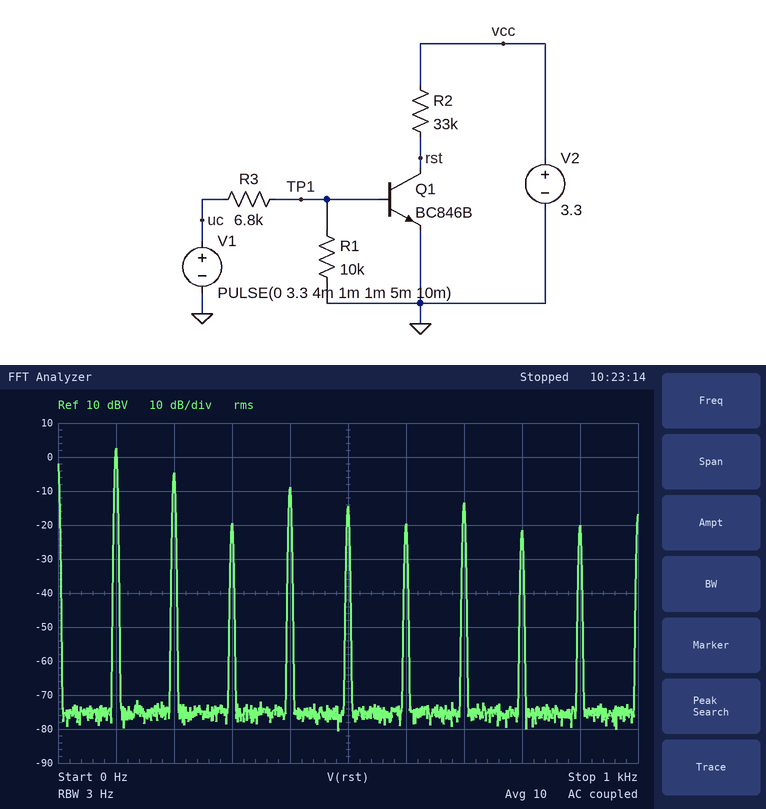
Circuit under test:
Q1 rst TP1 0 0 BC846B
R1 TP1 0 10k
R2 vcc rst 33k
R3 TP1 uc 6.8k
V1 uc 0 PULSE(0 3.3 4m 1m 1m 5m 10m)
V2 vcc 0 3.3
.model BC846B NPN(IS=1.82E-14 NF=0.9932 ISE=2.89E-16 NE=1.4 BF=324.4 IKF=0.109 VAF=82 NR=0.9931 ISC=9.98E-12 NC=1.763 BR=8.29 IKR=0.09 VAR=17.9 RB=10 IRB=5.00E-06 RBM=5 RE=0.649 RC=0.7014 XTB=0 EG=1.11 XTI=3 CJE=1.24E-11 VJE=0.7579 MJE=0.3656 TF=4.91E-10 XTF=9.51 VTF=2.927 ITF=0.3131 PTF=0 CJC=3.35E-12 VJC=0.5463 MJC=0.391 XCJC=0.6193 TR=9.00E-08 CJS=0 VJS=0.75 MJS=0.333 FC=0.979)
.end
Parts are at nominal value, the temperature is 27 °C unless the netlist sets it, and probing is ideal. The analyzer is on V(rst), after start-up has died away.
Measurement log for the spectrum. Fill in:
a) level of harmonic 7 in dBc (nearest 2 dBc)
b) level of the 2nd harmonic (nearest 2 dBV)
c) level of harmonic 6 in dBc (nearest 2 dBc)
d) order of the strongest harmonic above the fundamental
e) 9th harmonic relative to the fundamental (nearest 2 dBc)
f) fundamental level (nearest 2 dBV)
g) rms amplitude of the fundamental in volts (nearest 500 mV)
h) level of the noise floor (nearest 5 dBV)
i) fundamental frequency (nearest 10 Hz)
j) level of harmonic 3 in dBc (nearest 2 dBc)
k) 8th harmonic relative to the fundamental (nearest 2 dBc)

-16 dBc
-4 dBV
-22 dBc
2
-22 dBc
2 dBV
1.5 V
-75 dBV
100 Hz
-22 dBc
-24 dBc
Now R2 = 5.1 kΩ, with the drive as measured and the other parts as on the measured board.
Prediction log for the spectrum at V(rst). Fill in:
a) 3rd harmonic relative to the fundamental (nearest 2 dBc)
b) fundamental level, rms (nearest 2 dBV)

-20 dBc
2 dBV
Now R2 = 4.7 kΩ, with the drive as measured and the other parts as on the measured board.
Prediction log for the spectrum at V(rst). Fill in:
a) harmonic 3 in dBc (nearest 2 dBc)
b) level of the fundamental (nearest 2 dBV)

-20 dBc
2 dBV
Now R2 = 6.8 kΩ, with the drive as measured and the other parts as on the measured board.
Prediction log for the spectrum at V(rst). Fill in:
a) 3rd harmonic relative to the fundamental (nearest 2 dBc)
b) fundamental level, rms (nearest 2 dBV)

-20 dBc
2 dBV
